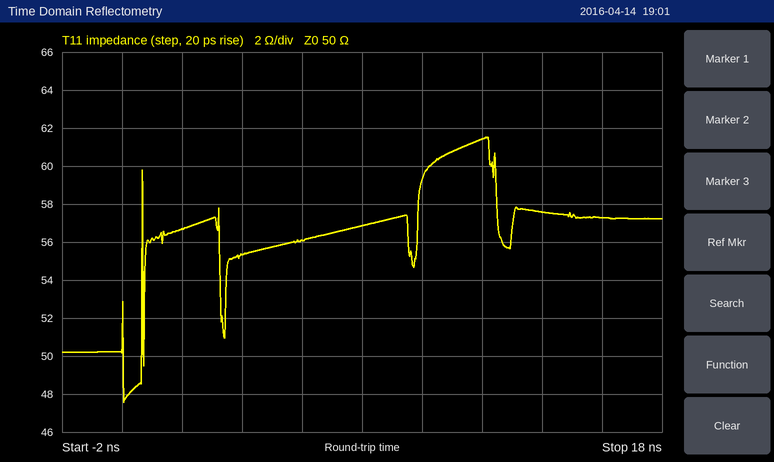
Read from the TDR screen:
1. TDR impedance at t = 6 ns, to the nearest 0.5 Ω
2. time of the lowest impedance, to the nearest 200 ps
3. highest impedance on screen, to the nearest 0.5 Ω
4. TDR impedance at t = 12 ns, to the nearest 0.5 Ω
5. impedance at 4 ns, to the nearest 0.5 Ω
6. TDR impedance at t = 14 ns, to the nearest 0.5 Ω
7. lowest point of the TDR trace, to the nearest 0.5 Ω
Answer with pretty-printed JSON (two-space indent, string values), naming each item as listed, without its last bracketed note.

{
  "TDR impedance at t = 6 ns, to the nearest 0.5 Ω": "56.0 Ω",
  "time of the lowest impedance, to the nearest 200 ps": "0.0 ns",
  "highest impedance on screen, to the nearest 0.5 Ω": "61.5 Ω",
  "TDR impedance at t = 12 ns, to the nearest 0.5 Ω": "61.5 Ω",
  "impedance at 4 ns, to the nearest 0.5 Ω": "55.5 Ω",
  "TDR impedance at t = 14 ns, to the nearest 0.5 Ω": "57.5 Ω",
  "lowest point of the TDR trace, to the nearest 0.5 Ω": "47.5 Ω"
}
